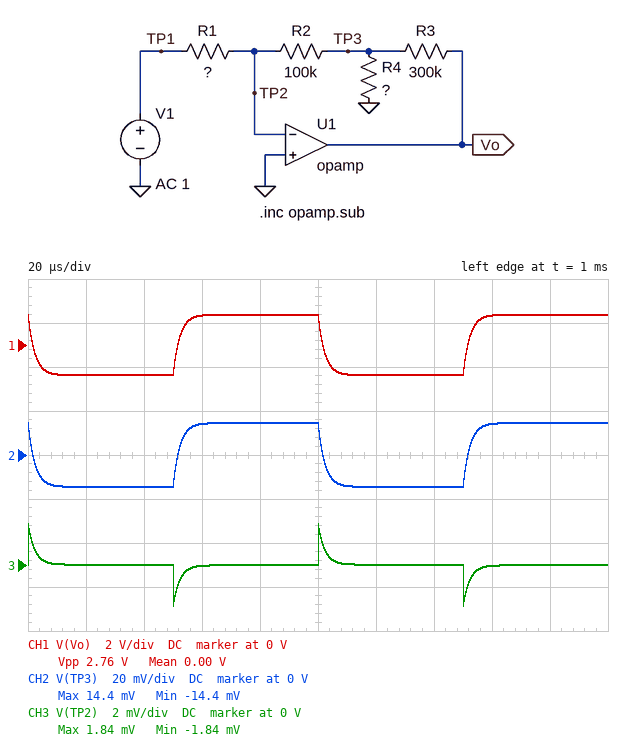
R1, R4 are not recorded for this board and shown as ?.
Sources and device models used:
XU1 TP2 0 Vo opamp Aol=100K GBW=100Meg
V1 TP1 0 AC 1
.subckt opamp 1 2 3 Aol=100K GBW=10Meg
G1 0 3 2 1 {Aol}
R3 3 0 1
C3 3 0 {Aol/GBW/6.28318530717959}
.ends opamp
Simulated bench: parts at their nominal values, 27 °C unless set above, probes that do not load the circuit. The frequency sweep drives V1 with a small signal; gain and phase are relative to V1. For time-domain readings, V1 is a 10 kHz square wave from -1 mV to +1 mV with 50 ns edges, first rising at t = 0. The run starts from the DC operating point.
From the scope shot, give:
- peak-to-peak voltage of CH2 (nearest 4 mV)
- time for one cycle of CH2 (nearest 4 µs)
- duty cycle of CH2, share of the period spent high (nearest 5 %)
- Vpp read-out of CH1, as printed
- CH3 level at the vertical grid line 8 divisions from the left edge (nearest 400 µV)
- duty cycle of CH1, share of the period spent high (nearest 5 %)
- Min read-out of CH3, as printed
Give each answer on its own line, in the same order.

28 mV
100 µs
50 %
2.76 V
0 V
50 %
-1.84 mV
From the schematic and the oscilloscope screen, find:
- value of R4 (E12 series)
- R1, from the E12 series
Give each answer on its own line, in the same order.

3.3 kΩ
6.8 kΩ
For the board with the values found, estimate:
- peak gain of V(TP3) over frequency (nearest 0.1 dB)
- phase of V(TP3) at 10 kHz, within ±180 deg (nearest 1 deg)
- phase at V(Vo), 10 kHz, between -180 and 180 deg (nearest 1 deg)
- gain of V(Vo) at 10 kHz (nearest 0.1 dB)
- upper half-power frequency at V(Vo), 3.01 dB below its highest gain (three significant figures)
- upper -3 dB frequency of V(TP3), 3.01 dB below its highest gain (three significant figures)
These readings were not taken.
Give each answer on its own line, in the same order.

23.2 dB
172 deg
172 deg
62.7 dB
68.2 kHz
68.2 kHz
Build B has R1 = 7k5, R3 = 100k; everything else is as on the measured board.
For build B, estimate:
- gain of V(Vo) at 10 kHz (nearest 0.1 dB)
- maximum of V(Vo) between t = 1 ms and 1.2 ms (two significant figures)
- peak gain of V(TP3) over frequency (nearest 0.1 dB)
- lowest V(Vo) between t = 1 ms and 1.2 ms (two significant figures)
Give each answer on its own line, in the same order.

52.6 dB
430 mV
22.5 dB
-430 mV
